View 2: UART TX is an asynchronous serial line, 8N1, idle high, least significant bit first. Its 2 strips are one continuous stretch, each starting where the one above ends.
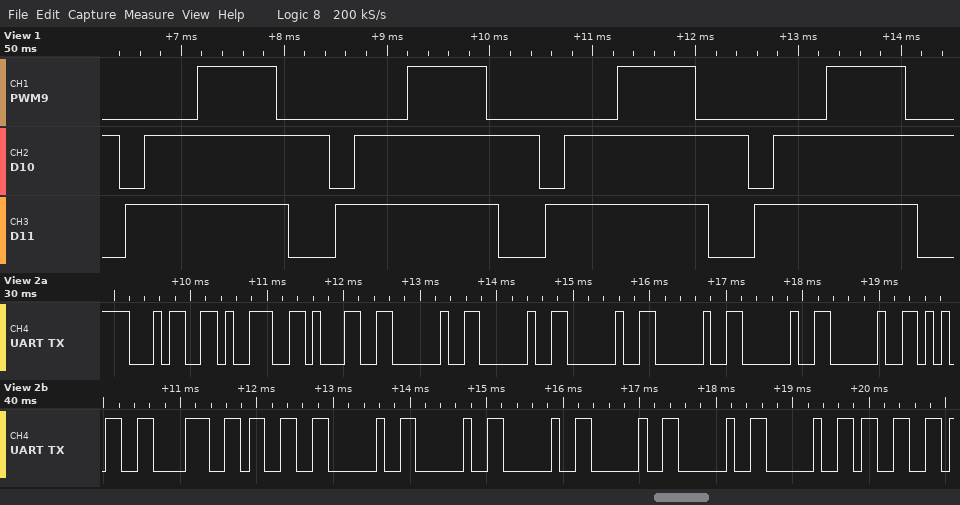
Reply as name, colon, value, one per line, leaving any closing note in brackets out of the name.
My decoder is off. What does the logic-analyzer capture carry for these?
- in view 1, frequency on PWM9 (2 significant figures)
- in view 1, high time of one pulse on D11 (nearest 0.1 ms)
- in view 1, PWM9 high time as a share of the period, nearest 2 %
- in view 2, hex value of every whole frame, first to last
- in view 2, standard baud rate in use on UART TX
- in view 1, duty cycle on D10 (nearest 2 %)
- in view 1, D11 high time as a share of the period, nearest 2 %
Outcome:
in view 1, frequency on PWM9: 490 Hz
in view 1, high time of one pulse on D11: 1.6 ms
in view 1, PWM9 high time as a share of the period, nearest 2 %: 38 %
in view 2, hex value of every whole frame, first to last: 34 39 31 20 20 20 20 20 20 35 38 33 20 20 20 20 20 20 33
in view 2, standard baud rate in use on UART TX: 9600 baud
in view 1, duty cycle on D10: 88 %
in view 1, D11 high time as a share of the period, nearest 2 %: 78 %
